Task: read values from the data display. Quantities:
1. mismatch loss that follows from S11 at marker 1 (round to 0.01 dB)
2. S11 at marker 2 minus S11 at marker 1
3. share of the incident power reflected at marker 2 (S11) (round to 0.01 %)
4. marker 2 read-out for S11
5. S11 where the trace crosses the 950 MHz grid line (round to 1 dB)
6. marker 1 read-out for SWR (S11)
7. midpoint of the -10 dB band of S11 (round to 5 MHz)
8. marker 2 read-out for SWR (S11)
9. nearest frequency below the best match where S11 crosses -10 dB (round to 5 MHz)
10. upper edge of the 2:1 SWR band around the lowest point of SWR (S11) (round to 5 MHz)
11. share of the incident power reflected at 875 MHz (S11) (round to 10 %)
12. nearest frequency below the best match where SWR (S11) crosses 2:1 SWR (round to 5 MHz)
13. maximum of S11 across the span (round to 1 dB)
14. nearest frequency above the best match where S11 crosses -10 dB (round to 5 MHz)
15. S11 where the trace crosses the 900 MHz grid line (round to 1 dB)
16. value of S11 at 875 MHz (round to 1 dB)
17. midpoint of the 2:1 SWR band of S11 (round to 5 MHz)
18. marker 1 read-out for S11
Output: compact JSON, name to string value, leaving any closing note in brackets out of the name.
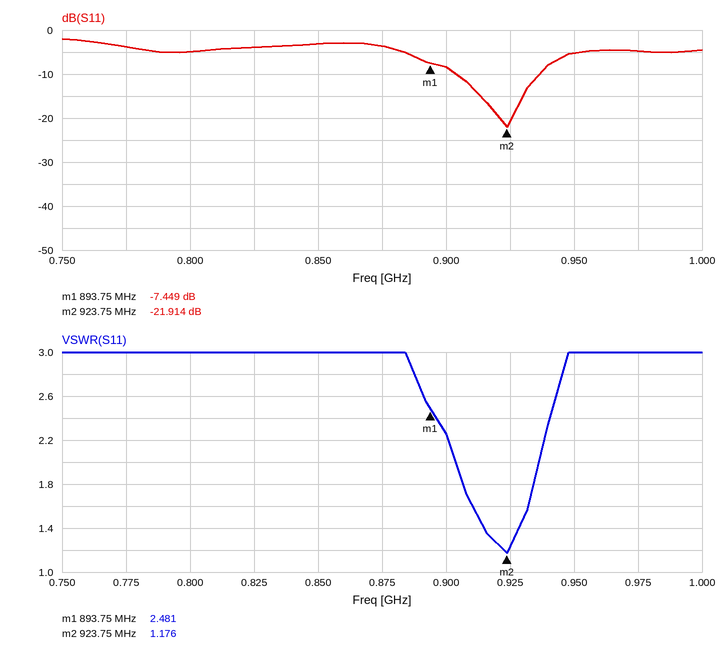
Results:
{"mismatch loss that follows from S11 at marker 1": "0.86 dB", "S11 at marker 2 minus S11 at marker 1": "-14.465 dB", "share of the incident power reflected at marker 2 (S11)": "0.64 %", "marker 2 read-out for S11": "-21.914 dB", "S11 where the trace crosses the 950 MHz grid line": "-5 dB", "marker 1 read-out for SWR": "2.481", "midpoint of the -10 dB band of S11": "920 MHz", "marker 2 read-out for SWR": "1.176", "nearest frequency below the best match where S11 crosses -10 dB": "905 MHz", "upper edge of the 2:1 SWR band around the lowest point of SWR (S11)": "935 MHz", "share of the incident power reflected at 875 MHz (S11)": "40 %", "nearest frequency below the best match where SWR (S11) crosses 2:1 SWR": "905 MHz", "maximum of S11 across the span": "-2 dB", "nearest frequency above the best match where S11 crosses -10 dB": "935 MHz", "S11 where the trace crosses the 900 MHz grid line": "-8 dB", "value of S11 at 875 MHz": "-4 dB", "midpoint of the 2:1 SWR band of S11": "920 MHz", "marker 1 read-out for S11": "-7.449 dB"}
